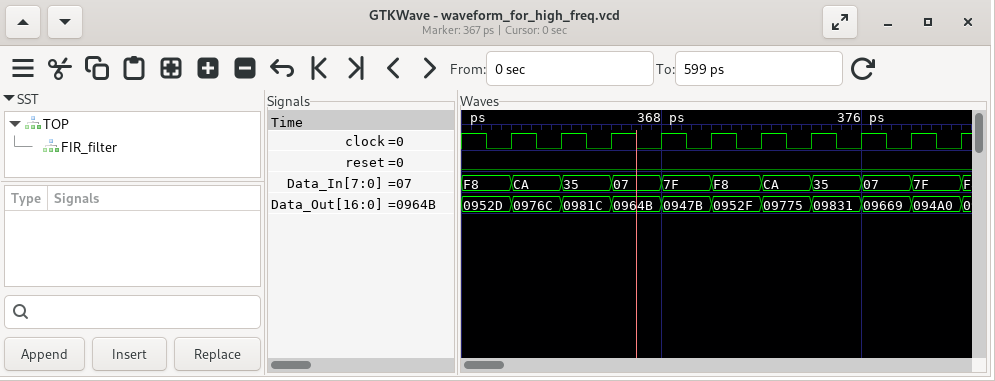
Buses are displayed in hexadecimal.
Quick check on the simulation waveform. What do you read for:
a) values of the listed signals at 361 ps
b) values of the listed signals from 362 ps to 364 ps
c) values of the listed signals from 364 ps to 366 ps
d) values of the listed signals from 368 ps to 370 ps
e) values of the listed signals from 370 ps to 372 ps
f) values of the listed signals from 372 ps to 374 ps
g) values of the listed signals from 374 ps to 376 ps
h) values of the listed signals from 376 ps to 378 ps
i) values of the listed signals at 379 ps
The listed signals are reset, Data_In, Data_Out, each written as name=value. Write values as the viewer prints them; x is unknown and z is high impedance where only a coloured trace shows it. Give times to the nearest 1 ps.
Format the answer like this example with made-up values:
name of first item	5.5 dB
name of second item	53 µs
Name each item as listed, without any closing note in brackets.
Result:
values of the listed signals at 361 ps	reset=0, Data_In=F8, Data_Out=0952D
values of the listed signals from 362 ps to 364 ps	reset=0, Data_In=CA, Data_Out=0976C
values of the listed signals from 364 ps to 366 ps	reset=0, Data_In=35, Data_Out=0981C
values of the listed signals from 368 ps to 370 ps	reset=0, Data_In=7F, Data_Out=0947B
values of the listed signals from 370 ps to 372 ps	reset=0, Data_In=F8, Data_Out=0952F
values of the listed signals from 372 ps to 374 ps	reset=0, Data_In=CA, Data_Out=09775
values of the listed signals from 374 ps to 376 ps	reset=0, Data_In=35, Data_Out=09831
values of the listed signals from 376 ps to 378 ps	reset=0, Data_In=07, Data_Out=09669
values of the listed signals at 379 ps	reset=0, Data_In=7F, Data_Out=094A0
